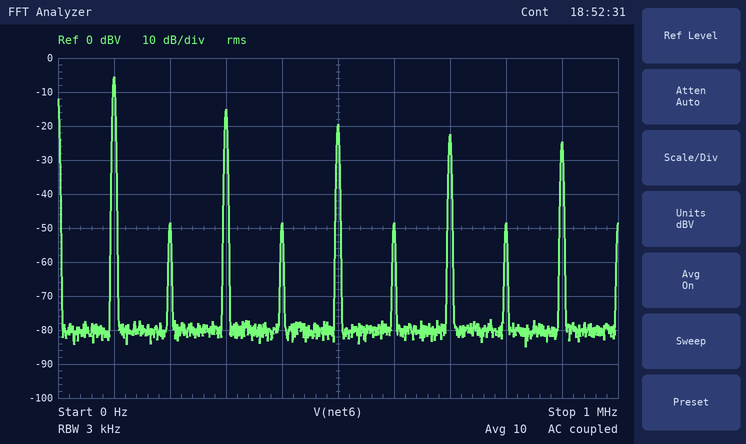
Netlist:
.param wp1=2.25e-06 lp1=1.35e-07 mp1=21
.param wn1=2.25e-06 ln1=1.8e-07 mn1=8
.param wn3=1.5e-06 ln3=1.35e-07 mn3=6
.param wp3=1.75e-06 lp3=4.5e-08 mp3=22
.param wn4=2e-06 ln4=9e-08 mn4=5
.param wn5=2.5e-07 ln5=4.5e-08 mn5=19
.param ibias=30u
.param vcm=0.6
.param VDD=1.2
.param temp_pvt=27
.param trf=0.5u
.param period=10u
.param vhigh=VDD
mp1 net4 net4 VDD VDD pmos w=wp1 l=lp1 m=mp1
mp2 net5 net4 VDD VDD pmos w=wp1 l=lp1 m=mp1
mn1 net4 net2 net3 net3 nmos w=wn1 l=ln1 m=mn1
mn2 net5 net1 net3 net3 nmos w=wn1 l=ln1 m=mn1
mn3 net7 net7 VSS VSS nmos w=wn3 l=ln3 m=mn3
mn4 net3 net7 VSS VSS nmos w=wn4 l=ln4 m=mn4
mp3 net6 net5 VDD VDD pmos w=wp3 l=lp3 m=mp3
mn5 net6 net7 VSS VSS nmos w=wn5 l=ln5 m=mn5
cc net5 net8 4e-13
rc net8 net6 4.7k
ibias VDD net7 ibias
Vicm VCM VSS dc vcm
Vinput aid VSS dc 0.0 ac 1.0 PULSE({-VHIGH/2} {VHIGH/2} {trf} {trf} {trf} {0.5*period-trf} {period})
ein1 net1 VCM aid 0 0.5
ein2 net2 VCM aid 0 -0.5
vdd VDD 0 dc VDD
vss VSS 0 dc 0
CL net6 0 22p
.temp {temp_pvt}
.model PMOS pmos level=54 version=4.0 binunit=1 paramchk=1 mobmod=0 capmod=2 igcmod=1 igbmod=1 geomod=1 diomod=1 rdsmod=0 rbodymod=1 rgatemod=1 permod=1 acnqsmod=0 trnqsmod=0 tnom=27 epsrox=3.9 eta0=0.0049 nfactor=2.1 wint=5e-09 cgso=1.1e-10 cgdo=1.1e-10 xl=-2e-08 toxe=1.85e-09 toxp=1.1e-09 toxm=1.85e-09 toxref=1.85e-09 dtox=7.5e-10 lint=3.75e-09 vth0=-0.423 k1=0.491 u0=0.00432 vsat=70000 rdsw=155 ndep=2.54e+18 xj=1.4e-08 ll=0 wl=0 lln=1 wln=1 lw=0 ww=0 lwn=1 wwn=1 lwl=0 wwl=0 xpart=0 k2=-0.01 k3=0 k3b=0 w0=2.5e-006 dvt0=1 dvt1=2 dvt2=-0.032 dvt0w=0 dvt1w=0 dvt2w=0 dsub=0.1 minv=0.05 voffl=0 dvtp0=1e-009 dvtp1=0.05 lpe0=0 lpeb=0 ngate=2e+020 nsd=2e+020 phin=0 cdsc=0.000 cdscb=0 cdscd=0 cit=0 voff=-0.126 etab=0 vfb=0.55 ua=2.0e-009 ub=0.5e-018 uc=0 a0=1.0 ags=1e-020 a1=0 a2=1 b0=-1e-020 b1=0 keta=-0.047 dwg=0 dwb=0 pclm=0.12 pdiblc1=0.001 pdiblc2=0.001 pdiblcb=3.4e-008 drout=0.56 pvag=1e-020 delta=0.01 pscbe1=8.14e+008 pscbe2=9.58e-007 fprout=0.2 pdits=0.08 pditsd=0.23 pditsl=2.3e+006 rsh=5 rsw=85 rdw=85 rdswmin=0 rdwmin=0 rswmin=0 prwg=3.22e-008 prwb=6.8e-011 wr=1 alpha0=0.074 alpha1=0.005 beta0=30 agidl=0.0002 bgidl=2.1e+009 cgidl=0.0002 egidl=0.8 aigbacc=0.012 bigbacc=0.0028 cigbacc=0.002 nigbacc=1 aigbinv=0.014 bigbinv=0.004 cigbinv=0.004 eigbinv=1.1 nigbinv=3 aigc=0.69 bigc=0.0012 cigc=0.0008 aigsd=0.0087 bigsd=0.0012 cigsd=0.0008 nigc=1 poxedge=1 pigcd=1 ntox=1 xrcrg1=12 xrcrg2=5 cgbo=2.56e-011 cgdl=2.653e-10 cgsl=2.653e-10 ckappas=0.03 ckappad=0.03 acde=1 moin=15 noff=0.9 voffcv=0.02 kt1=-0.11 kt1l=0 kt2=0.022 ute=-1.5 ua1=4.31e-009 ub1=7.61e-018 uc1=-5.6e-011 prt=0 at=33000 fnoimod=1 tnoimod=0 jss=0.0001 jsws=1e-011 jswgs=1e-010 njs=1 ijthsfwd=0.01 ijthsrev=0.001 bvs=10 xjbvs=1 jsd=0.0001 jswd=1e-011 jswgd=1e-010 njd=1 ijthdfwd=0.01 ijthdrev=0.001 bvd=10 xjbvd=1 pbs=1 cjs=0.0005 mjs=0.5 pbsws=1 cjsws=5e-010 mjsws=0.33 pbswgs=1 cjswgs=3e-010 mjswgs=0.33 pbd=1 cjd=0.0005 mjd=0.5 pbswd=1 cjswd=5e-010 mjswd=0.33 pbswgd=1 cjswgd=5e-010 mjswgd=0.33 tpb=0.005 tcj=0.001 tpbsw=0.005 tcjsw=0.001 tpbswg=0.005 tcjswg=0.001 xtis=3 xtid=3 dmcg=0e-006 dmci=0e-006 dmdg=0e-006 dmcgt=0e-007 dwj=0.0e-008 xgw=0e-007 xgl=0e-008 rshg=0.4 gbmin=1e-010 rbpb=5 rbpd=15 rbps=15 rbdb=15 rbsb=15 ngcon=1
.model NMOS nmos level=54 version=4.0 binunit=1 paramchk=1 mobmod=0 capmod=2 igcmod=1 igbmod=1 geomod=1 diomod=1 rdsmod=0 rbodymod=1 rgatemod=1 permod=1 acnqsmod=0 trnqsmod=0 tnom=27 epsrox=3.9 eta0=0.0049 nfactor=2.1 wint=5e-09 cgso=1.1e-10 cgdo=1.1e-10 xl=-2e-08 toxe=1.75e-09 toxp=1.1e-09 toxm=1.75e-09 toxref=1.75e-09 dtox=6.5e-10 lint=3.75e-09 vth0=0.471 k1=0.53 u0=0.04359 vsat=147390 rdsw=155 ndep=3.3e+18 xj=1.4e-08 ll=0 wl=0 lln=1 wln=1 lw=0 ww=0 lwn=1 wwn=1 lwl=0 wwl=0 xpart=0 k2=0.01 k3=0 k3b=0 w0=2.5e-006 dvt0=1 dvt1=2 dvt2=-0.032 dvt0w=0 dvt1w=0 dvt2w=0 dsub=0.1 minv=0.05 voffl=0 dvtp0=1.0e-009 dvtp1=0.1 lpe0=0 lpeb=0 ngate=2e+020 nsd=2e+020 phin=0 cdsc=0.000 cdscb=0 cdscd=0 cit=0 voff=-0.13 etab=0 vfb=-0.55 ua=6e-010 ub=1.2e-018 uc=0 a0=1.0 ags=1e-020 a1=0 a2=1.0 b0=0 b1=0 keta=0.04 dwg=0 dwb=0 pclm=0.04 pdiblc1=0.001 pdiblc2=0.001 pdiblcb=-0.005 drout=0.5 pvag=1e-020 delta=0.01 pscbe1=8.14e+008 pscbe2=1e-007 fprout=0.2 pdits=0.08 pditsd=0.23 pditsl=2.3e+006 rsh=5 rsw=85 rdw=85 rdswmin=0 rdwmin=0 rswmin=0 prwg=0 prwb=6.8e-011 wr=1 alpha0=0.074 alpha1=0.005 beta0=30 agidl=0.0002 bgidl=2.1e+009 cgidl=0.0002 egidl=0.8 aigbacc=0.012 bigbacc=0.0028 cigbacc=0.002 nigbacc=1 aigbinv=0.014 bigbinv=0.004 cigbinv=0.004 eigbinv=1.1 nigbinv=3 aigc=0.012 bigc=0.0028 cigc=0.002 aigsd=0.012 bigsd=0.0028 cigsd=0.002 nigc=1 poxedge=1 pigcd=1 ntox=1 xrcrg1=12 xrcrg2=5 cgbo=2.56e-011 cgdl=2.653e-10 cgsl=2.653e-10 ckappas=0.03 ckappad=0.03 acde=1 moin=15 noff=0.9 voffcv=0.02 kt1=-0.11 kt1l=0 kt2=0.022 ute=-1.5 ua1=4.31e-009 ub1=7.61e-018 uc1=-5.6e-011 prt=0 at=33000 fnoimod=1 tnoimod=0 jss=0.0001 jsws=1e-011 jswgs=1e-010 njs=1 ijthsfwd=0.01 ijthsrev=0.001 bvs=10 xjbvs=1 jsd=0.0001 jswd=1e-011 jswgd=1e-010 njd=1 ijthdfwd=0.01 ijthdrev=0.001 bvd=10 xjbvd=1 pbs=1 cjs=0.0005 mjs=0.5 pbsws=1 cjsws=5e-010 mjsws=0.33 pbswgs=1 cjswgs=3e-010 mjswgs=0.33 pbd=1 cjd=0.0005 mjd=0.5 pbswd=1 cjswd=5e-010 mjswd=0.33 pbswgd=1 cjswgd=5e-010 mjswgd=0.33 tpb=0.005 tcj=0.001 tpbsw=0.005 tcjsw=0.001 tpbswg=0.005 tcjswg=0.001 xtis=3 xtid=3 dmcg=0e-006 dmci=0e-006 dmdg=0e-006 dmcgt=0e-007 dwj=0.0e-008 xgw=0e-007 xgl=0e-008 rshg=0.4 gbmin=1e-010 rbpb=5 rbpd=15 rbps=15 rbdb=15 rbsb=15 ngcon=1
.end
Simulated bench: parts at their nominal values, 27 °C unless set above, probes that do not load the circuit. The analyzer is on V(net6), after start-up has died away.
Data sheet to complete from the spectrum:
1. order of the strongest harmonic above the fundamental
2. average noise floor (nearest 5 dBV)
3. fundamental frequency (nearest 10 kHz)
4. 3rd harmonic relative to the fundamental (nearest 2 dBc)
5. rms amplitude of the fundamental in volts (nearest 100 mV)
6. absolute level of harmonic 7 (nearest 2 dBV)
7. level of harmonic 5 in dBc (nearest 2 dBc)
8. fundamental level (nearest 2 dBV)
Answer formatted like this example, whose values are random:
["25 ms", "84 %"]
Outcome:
["3", "-80 dBV", "100 kHz", "-10 dBc", "500 mV", "-22 dBV", "-14 dBc", "-6 dBV"]
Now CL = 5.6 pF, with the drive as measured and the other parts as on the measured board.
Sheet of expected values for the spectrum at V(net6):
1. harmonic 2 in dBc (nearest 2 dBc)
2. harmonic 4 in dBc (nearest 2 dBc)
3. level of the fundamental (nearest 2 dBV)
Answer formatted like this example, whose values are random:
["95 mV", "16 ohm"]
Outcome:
["-54 dBc", "-54 dBc", "-6 dBV"]
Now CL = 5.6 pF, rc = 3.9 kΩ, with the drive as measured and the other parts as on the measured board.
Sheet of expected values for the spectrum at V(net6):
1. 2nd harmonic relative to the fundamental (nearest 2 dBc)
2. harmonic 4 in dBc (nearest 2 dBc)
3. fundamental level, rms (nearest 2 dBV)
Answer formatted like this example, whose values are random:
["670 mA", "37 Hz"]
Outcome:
["-54 dBc", "-54 dBc", "-6 dBV"]
